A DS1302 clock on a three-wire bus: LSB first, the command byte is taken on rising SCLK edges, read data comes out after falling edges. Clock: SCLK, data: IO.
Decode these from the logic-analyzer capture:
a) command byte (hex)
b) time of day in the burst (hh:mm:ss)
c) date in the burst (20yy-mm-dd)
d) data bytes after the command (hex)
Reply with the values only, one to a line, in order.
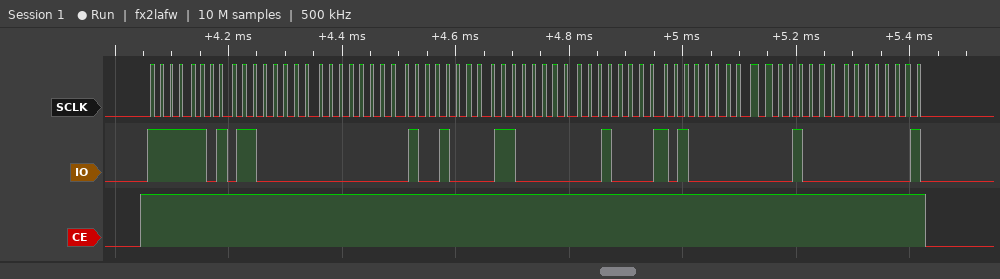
0xBF
12:00:06
2010-08-06
06 00 12 06 08 05 10 80
